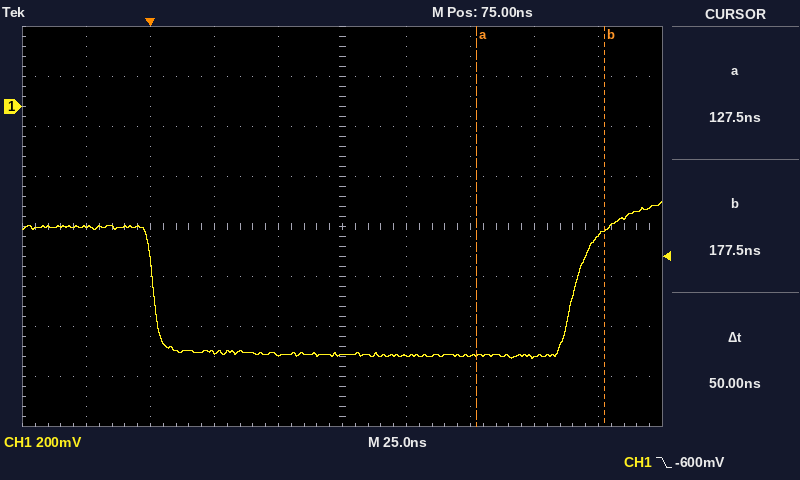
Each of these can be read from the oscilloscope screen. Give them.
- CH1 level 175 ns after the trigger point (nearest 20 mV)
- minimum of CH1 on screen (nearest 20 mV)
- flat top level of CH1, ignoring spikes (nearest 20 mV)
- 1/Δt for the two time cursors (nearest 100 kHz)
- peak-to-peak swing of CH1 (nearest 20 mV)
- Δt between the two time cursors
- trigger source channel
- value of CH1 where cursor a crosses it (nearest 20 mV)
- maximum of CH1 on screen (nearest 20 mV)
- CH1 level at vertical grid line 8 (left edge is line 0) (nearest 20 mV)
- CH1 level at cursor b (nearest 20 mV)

-520 mV
-1.00 V
-480 mV
20.0 MHz
620 mV
50 ns
CH1
-1.00 V
-380 mV
-1.00 V
-500 mV
